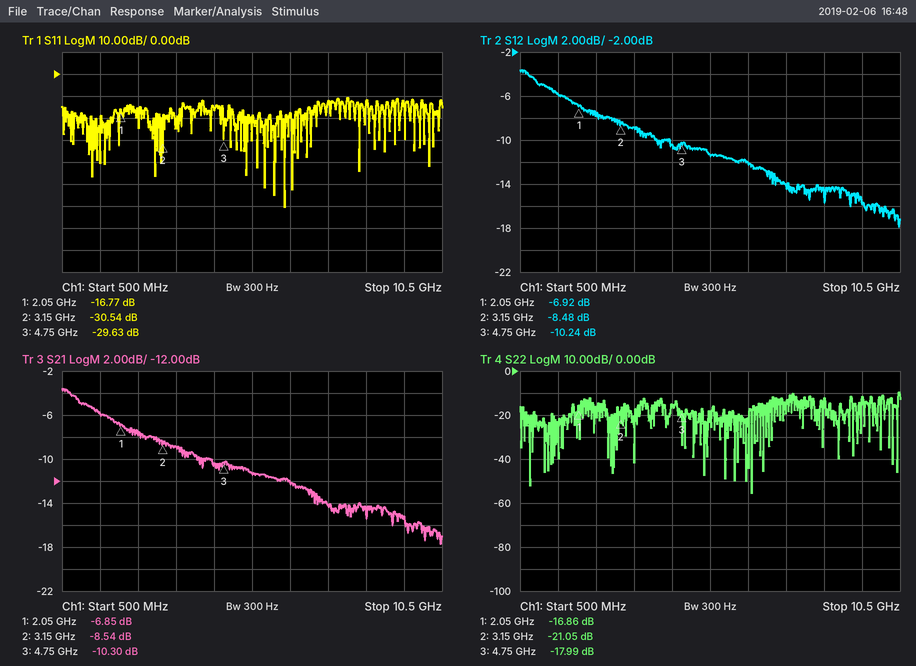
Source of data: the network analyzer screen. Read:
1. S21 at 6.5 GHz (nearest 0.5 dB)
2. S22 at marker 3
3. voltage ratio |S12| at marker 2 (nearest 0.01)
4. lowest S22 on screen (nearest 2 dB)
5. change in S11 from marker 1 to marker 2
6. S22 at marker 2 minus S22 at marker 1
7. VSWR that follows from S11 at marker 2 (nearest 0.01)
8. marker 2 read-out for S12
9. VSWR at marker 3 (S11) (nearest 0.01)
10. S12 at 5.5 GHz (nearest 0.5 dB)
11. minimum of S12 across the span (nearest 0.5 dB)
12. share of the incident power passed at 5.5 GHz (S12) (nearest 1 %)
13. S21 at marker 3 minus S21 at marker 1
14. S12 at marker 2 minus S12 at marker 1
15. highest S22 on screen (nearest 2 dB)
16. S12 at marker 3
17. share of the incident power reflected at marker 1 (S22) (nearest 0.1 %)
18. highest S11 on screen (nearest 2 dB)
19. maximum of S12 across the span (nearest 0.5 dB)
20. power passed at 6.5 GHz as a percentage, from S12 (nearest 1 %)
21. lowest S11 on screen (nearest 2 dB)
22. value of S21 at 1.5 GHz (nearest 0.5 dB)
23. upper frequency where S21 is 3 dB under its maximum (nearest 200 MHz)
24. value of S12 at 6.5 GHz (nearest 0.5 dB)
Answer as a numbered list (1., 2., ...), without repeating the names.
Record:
1. -12.0 dB
2. -17.99 dB
3. 0.38
4. -56 dB
5. -13.77 dB
6. -4.19 dB
7. 1.06
8. -8.48 dB
9. 1.07
10. -11.5 dB
11. -18.0 dB
12. 7 %
13. -3.45 dB
14. -1.56 dB
15. -10 dB
16. -10.24 dB
17. 2.1 %
18. -10 dB
19. -3.5 dB
20. 6 %
21. -60 dB
22. -6.0 dB
23. 1.8 GHz
24. -12.0 dB
